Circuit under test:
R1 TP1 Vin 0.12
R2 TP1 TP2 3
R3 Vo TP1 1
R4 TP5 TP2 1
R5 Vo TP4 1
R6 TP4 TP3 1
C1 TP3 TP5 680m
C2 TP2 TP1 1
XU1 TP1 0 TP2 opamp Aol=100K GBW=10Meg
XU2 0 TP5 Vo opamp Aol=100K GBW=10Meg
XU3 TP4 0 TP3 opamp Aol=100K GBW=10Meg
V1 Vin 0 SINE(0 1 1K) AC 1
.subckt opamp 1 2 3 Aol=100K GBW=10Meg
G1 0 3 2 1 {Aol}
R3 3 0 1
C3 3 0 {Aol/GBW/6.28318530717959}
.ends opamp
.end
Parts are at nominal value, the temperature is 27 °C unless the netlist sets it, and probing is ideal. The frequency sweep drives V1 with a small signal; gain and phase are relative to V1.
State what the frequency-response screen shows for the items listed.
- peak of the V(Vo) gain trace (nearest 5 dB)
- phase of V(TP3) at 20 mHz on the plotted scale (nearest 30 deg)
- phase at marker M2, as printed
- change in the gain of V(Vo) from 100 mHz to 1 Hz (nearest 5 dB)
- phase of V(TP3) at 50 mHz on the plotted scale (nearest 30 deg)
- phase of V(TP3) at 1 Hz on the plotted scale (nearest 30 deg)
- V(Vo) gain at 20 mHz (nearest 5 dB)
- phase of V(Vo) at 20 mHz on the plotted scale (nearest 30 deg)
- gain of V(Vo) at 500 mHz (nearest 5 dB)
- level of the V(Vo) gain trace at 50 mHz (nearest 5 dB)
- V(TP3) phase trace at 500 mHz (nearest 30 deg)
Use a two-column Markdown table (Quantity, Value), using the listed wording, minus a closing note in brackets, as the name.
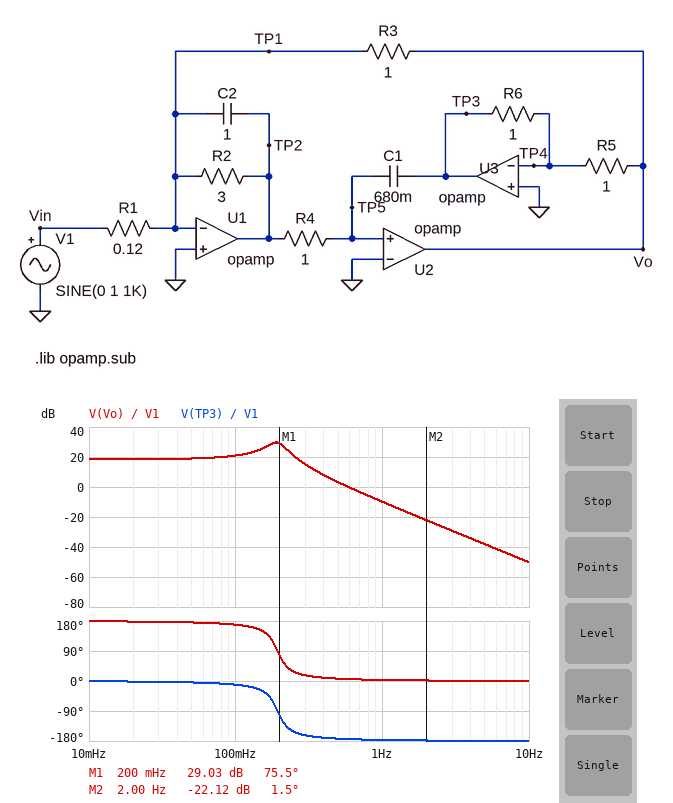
| Quantity | Value |
|---|---|
| peak of the V(Vo) gain trace | 30 dB |
| phase of V(TP3) at 20 mHz on the plotted scale | 0 deg |
| phase at marker M2, as printed | 1.5 deg |
| change in the gain of V(Vo) from 100 mHz to 1 Hz | -30 dB |
| phase of V(TP3) at 50 mHz on the plotted scale | 0 deg |
| phase of V(TP3) at 1 Hz on the plotted scale | -180 deg |
| V(Vo) gain at 20 mHz | 20 dB |
| phase of V(Vo) at 20 mHz on the plotted scale | 180 deg |
| gain of V(Vo) at 500 mHz | 5 dB |
| level of the V(Vo) gain trace at 50 mHz | 20 dB |
| V(TP3) phase trace at 500 mHz | -180 deg |
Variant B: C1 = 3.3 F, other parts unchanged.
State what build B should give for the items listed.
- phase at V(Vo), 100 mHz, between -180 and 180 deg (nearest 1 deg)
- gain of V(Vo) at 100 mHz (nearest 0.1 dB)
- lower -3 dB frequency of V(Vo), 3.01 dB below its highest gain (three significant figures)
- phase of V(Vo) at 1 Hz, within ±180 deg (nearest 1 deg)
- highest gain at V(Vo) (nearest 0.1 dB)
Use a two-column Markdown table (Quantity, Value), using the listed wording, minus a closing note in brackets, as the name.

| Quantity | Value |
|---|---|
| phase at V(Vo), 100 mHz, between -180 and 180 deg | 66 deg |
| gain of V(Vo) at 100 mHz | 20.9 dB |
| lower -3 dB frequency of V(Vo), 3.01 dB below its highest gain | 42.8 mHz |
| phase of V(Vo) at 1 Hz, within ±180 deg | 3 deg |
| highest gain at V(Vo) | 23.2 dB |
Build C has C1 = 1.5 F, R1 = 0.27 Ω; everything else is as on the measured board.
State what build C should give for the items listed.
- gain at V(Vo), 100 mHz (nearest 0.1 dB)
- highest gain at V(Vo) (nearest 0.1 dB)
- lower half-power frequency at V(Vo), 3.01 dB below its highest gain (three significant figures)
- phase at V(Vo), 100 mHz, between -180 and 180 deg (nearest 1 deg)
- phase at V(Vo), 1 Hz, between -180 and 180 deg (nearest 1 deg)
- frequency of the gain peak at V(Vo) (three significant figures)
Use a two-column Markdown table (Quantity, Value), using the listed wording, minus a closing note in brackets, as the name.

| Quantity | Value |
|---|---|
| gain at V(Vo), 100 mHz | 17.1 dB |
| highest gain at V(Vo) | 19.3 dB |
| lower half-power frequency at V(Vo), 3.01 dB below its highest gain | 93.4 mHz |
| phase at V(Vo), 100 mHz, between -180 and 180 deg | 142 deg |
| phase at V(Vo), 1 Hz, between -180 and 180 deg | 3 deg |
| frequency of the gain peak at V(Vo) | 124 mHz |
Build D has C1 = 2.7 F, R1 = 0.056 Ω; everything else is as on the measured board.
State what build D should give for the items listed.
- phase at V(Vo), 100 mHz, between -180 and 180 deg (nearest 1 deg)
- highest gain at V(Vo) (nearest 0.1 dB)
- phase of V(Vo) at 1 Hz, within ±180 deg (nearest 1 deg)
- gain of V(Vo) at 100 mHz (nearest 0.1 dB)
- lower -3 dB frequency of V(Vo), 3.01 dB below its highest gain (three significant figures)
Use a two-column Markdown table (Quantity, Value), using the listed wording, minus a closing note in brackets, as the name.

| Quantity | Value |
|---|---|
| phase at V(Vo), 100 mHz, between -180 and 180 deg | 83 deg |
| highest gain at V(Vo) | 30.6 dB |
| phase of V(Vo) at 1 Hz, within ±180 deg | 3 deg |
| gain of V(Vo) at 100 mHz | 29.9 dB |
| lower -3 dB frequency of V(Vo), 3.01 dB below its highest gain | 55.0 mHz |
